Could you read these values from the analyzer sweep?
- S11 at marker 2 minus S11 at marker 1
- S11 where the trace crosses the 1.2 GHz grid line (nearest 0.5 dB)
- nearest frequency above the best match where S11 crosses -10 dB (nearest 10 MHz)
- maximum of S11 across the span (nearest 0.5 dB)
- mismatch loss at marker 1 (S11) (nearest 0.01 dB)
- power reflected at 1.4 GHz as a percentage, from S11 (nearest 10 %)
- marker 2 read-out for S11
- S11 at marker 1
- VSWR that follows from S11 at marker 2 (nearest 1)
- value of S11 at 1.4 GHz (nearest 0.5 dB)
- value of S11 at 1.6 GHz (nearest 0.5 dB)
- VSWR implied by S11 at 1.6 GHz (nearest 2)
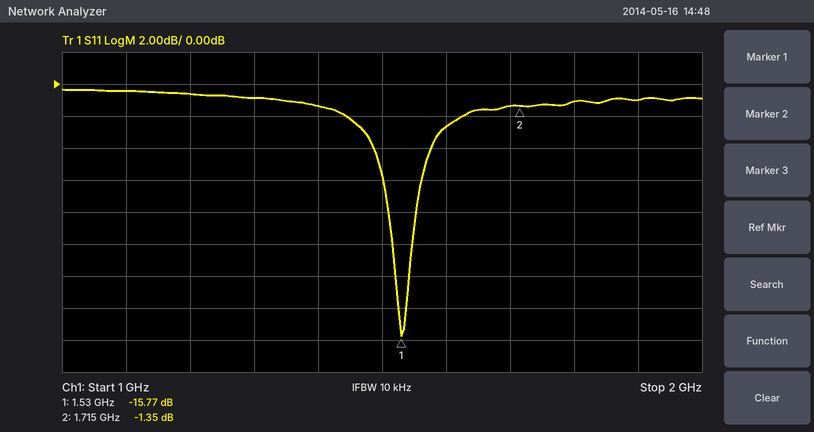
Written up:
14.42 dB
-0.5 dB
1.55 GHz
-0.5 dB
0.12 dB
70 %
-1.35 dB
-15.77 dB
13
-1.5 dB
-2.5 dB
6
